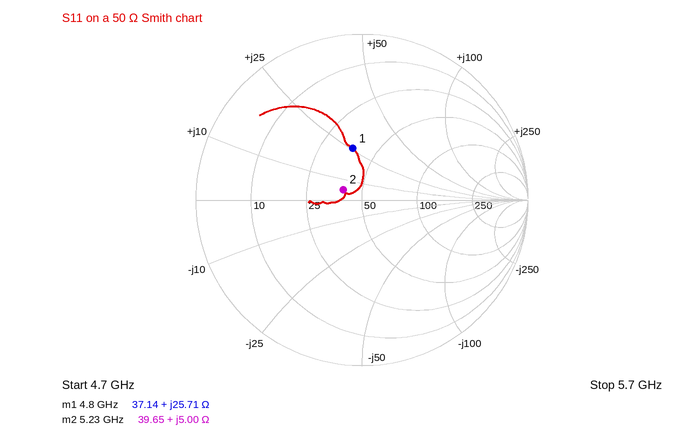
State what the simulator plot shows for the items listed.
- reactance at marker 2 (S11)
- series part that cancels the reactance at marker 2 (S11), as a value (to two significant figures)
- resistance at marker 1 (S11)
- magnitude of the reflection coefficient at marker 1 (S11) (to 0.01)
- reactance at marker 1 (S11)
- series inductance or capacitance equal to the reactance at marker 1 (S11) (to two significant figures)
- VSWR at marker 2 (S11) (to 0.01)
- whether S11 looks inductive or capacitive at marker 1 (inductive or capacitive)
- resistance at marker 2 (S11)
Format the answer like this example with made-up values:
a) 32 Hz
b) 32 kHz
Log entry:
a) +5.00 Ω
b) 6.1 pF
c) 37.14 Ω
d) 0.32
e) +25.71 Ω
f) 850 pH
g) 1.29
h) inductive
i) 39.65 Ω
